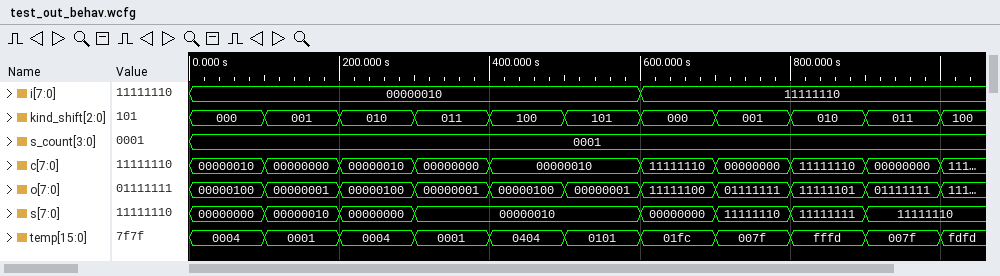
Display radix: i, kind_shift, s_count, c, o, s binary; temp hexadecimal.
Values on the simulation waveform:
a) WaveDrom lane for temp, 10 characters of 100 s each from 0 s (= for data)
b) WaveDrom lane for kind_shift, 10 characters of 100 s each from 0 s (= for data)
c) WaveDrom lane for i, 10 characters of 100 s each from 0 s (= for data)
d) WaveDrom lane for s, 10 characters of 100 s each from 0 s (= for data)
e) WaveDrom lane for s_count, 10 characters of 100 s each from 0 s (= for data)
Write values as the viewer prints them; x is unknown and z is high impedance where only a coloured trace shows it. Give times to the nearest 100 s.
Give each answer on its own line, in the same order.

{name: 'temp', wave: '==========', data: '0004 0001 0004 0001 0404 0101 01fc 007f fffd 007f'}
{name: 'kind_shift', wave: '==========', data: '000 001 010 011 100 101 000 001 010 011'}
{name: 'i', wave: '=.....=...', data: '00000010 11111110'}
{name: 's', wave: '====..====', data: '00000000 00000010 00000000 00000010 00000000 11111110 11111111 11111110'}
{name: 's_count', wave: '=.........', data: '0001'}
